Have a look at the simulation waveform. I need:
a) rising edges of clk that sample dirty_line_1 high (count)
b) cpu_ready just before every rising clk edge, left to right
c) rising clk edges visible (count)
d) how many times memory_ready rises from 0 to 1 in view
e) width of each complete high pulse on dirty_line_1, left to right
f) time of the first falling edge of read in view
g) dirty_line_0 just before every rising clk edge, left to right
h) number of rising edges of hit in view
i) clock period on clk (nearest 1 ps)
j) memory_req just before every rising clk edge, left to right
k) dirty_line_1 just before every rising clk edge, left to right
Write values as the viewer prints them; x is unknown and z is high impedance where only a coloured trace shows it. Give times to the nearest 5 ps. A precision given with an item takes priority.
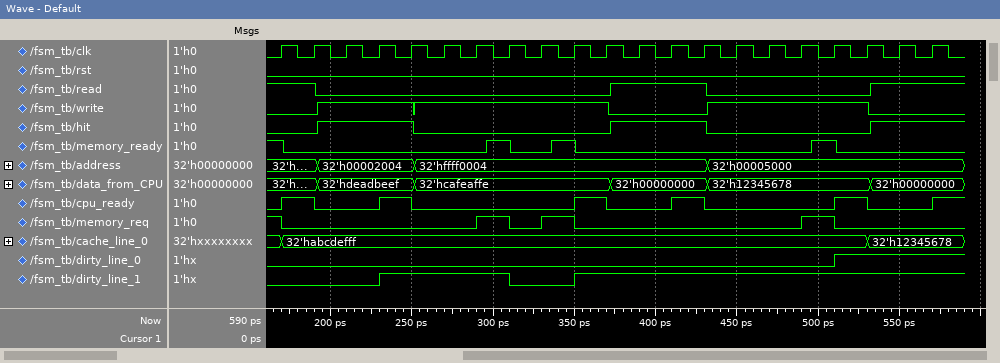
15
0 1 0 0 1 0 0 0 0 0 1 0 0 1 0 0 0 0 1 0 0
21
3
80 ps
190 ps
0 0 0 0 0 0 0 0 0 0 0 0 0 0 0 0 0 0 1 1 1
3
20 ps
1 0 0 0 0 0 0 1 0 1 0 0 0 0 0 0 0 1 0 0 0
0 0 0 0 1 1 1 1 0 0 1 1 1 1 1 1 1 1 1 1 1
